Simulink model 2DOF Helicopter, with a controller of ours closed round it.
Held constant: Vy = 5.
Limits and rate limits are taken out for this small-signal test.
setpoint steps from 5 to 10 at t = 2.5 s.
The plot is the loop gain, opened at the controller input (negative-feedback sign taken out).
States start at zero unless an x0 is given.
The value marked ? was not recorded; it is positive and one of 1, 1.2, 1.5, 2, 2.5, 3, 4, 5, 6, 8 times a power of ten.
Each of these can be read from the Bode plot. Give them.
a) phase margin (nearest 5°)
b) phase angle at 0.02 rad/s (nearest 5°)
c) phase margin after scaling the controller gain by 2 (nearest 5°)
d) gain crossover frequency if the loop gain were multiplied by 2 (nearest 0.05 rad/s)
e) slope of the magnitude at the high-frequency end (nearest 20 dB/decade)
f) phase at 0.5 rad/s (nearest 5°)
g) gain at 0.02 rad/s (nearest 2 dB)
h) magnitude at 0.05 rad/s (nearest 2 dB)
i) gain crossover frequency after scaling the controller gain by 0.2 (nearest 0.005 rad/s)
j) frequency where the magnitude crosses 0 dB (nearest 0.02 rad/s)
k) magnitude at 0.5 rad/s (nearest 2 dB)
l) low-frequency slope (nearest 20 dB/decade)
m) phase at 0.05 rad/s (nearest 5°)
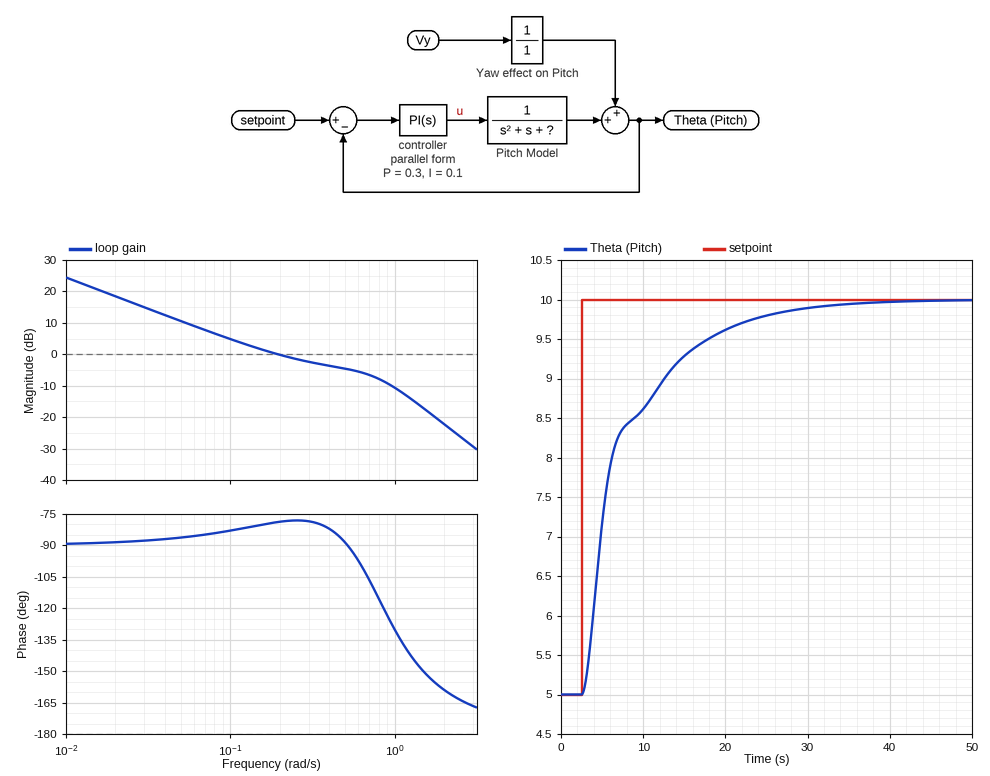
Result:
100°
-90°
80°
0.65 rad/s
-40 dB/decade
-90°
18 dB
10 dB
0.035 rad/s
0.20 rad/s
-4 dB
-20 dB/decade
-85°
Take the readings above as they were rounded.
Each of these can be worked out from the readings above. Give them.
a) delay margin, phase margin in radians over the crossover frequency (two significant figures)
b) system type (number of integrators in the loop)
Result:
8.7 s
1
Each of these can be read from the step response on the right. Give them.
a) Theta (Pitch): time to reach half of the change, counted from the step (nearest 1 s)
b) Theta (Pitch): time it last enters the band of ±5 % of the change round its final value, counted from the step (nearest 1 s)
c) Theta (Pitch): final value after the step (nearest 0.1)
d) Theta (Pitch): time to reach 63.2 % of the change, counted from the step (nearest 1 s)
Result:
3 s
21 s
10.0
4 s
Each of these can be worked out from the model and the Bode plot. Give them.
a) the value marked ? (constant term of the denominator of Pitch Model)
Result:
0.6
